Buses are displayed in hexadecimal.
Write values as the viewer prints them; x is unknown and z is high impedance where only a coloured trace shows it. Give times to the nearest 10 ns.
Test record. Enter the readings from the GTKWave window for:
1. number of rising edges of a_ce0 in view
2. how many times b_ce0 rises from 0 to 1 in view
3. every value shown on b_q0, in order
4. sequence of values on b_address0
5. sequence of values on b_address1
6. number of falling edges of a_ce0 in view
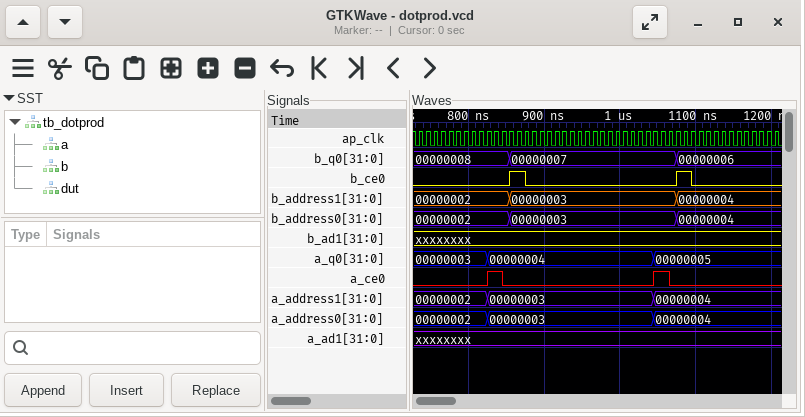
2
2
00000008, 00000007, 00000006
00000002, 00000003, 00000004
00000002, 00000003, 00000004
2
